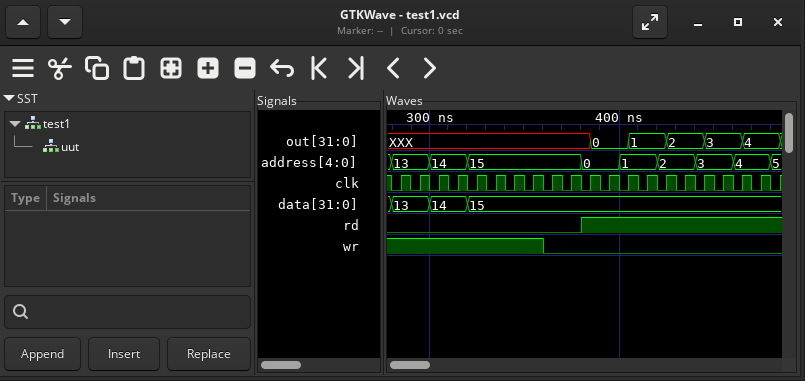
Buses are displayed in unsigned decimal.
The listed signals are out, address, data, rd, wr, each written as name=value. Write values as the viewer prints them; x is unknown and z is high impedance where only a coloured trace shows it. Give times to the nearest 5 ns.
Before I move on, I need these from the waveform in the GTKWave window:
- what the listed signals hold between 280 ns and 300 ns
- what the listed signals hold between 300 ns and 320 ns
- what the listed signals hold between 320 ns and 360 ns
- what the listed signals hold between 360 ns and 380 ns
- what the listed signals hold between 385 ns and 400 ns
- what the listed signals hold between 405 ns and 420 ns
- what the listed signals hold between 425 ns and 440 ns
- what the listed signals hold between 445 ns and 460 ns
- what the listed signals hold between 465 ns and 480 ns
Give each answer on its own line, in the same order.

out=XXX, address=13, data=13, rd=0, wr=1
out=XXX, address=14, data=14, rd=0, wr=1
out=XXX, address=15, data=15, rd=0, wr=1
out=XXX, address=15, data=15, rd=0, wr=0
out=0, address=0, data=15, rd=1, wr=0
out=1, address=1, data=15, rd=1, wr=0
out=2, address=2, data=15, rd=1, wr=0
out=3, address=3, data=15, rd=1, wr=0
out=4, address=4, data=15, rd=1, wr=0
